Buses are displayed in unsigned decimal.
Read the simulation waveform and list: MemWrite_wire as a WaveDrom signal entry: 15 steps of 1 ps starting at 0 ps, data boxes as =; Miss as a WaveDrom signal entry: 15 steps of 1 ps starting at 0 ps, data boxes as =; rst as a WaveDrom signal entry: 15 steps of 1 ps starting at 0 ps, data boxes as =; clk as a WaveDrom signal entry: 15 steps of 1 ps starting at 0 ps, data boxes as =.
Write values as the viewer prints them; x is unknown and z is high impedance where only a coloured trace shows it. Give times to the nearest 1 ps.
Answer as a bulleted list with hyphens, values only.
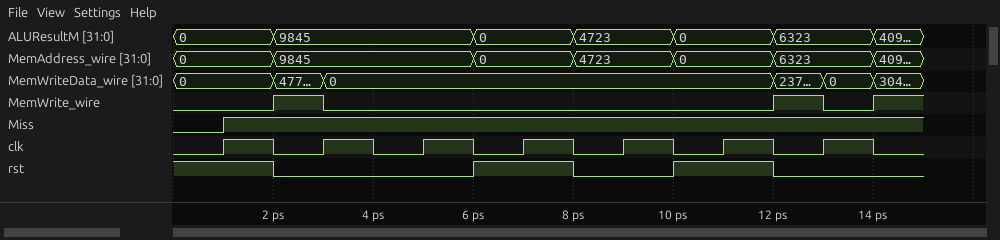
- {name: 'MemWrite_wire', wave: '0.10........101'}
- {name: 'Miss', wave: '01.............'}
- {name: 'rst', wave: '1.0...1.0.1.0..'}
- {name: 'clk', wave: '010101010101010'}
